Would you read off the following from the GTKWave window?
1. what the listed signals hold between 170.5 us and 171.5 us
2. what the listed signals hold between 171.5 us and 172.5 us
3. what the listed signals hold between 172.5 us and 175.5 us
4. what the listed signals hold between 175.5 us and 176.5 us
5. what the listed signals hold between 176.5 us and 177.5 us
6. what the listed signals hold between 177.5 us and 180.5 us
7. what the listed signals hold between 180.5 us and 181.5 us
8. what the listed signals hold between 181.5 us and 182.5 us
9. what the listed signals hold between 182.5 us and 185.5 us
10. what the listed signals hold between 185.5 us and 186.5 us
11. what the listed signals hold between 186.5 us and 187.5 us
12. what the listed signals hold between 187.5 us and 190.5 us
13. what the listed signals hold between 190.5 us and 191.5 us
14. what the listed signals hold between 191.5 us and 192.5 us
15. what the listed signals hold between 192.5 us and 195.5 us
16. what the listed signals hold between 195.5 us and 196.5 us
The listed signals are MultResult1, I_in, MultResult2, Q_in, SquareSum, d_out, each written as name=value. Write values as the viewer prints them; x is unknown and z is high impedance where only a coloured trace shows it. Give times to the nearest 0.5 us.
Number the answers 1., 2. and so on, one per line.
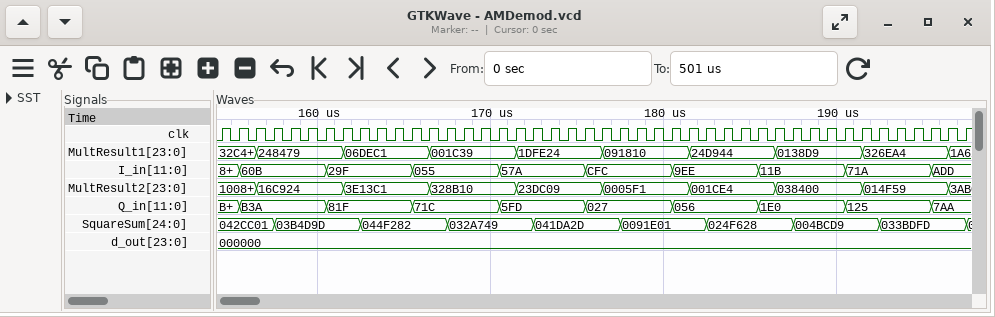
1. MultResult1=001C39, I_in=57A, MultResult2=328B10, Q_in=5FD, SquareSum=032A749, d_out=000000
2. MultResult1=1DFE24, I_in=57A, MultResult2=23DC09, Q_in=5FD, SquareSum=032A749, d_out=000000
3. MultResult1=1DFE24, I_in=57A, MultResult2=23DC09, Q_in=5FD, SquareSum=041DA2D, d_out=000000
4. MultResult1=1DFE24, I_in=CFC, MultResult2=23DC09, Q_in=027, SquareSum=041DA2D, d_out=000000
5. MultResult1=091810, I_in=CFC, MultResult2=0005F1, Q_in=027, SquareSum=041DA2D, d_out=000000
6. MultResult1=091810, I_in=CFC, MultResult2=0005F1, Q_in=027, SquareSum=0091E01, d_out=000000
7. MultResult1=091810, I_in=9EE, MultResult2=0005F1, Q_in=056, SquareSum=0091E01, d_out=000000
8. MultResult1=24D944, I_in=9EE, MultResult2=001CE4, Q_in=056, SquareSum=0091E01, d_out=000000
9. MultResult1=24D944, I_in=9EE, MultResult2=001CE4, Q_in=056, SquareSum=024F628, d_out=000000
10. MultResult1=24D944, I_in=11B, MultResult2=001CE4, Q_in=1E0, SquareSum=024F628, d_out=000000
11. MultResult1=0138D9, I_in=11B, MultResult2=038400, Q_in=1E0, SquareSum=024F628, d_out=000000
12. MultResult1=0138D9, I_in=11B, MultResult2=038400, Q_in=1E0, SquareSum=004BCD9, d_out=000000
13. MultResult1=0138D9, I_in=71A, MultResult2=038400, Q_in=125, SquareSum=004BCD9, d_out=000000
14. MultResult1=326EA4, I_in=71A, MultResult2=014F59, Q_in=125, SquareSum=004BCD9, d_out=000000
15. MultResult1=326EA4, I_in=71A, MultResult2=014F59, Q_in=125, SquareSum=033BDFD, d_out=000000
16. MultResult1=326EA4, I_in=ADD, MultResult2=014F59, Q_in=7AA, SquareSum=033BDFD, d_out=000000
